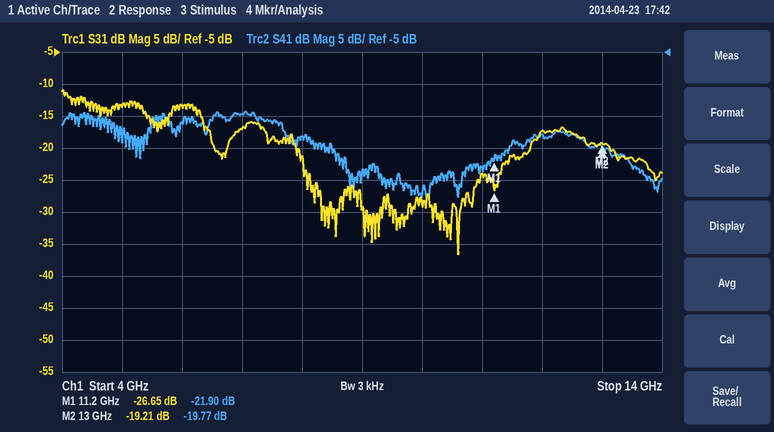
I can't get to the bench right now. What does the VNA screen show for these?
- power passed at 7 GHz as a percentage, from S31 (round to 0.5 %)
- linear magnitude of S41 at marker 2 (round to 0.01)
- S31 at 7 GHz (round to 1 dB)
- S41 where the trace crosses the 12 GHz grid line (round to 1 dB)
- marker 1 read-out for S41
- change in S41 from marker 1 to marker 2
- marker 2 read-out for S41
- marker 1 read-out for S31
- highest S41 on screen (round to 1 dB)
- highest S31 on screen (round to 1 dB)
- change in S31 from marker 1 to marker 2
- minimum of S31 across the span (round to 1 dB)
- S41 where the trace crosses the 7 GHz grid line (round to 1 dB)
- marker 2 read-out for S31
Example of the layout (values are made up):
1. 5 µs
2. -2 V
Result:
1. 2.0 %
2. 0.10
3. -17 dB
4. -18 dB
5. -21.90 dB
6. 2.13 dB
7. -19.77 dB
8. -26.65 dB
9. -14 dB
10. -11 dB
11. 7.44 dB
12. -37 dB
13. -15 dB
14. -19.21 dB
